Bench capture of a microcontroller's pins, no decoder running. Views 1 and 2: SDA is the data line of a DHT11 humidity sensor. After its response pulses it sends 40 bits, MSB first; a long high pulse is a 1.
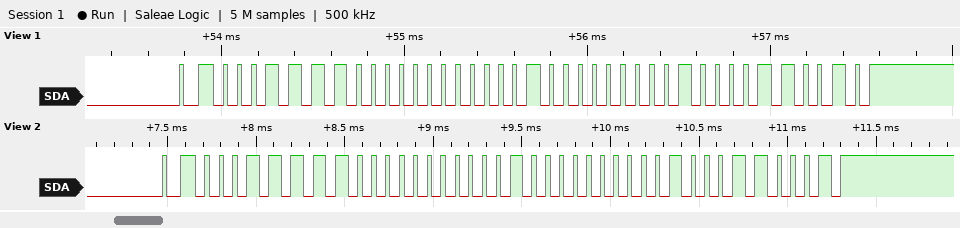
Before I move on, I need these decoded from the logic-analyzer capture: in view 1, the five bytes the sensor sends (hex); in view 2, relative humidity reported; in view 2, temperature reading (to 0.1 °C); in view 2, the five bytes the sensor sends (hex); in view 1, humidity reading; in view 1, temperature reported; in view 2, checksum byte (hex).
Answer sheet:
1E 00 10 04 32
31 %
16.2 °C
1F 00 10 02 31
30 %
16.4 °C
0x31
